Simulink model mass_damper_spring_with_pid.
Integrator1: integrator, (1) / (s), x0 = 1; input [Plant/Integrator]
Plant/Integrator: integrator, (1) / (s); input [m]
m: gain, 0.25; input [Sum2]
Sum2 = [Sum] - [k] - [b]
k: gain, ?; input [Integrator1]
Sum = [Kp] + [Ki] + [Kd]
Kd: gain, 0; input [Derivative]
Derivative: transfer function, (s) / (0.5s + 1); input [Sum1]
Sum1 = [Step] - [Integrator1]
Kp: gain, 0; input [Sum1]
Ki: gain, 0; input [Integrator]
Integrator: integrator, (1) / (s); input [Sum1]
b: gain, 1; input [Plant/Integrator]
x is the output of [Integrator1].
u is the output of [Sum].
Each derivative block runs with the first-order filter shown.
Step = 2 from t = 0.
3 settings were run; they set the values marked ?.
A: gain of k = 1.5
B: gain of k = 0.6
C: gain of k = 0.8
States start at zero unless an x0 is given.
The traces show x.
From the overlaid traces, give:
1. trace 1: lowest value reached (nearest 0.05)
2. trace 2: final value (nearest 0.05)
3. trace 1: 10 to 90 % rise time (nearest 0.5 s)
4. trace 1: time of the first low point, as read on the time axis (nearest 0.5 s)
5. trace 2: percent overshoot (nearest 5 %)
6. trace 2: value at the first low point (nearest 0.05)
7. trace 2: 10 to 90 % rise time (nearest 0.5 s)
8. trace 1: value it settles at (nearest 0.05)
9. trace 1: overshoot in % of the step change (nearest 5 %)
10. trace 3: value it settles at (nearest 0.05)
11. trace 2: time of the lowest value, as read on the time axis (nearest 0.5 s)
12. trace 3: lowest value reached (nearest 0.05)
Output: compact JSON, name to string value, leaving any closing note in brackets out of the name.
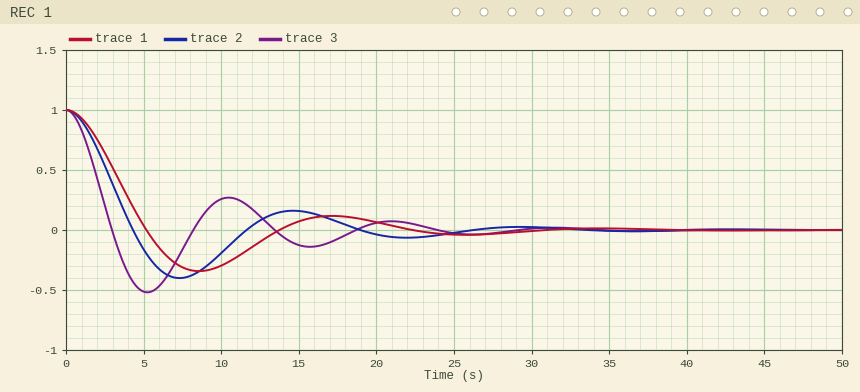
{"trace 1: lowest value reached": "-0.35", "trace 2: final value": "0.00", "trace 1: 10 to 90 % rise time": "3.5 s", "trace 1: time of the first low point, as read on the time axis": "8.5 s", "trace 2: percent overshoot": "40 %", "trace 2: value at the first low point": "-0.40", "trace 2: 10 to 90 % rise time": "3.0 s", "trace 1: value it settles at": "0.00", "trace 1: overshoot in % of the step change": "35 %", "trace 3: value it settles at": "0.00", "trace 2: time of the lowest value, as read on the time axis": "7.5 s", "trace 3: lowest value reached": "-0.50"}
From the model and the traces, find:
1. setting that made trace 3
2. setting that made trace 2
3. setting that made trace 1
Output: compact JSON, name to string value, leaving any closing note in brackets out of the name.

{"setting that made trace 3": "A", "setting that made trace 2": "C", "setting that made trace 1": "B"}
